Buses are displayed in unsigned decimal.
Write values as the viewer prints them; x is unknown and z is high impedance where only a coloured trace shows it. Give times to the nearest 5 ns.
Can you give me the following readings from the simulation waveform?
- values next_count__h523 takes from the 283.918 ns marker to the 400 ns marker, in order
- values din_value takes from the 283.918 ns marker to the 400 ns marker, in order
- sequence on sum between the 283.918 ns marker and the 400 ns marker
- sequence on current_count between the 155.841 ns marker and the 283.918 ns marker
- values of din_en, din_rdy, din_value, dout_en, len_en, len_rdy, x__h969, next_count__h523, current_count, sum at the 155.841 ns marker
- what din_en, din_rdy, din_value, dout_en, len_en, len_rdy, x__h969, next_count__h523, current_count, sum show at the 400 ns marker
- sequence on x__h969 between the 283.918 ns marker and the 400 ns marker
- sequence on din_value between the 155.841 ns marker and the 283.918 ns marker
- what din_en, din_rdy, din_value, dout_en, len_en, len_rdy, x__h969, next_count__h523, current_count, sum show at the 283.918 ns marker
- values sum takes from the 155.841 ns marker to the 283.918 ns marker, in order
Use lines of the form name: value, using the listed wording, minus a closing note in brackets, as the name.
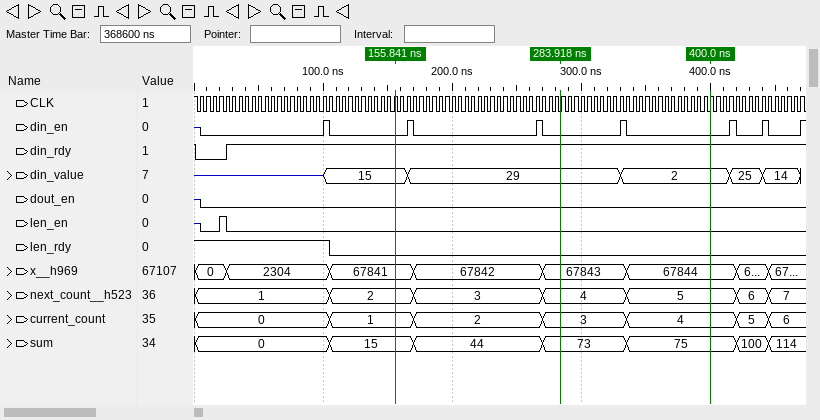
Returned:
values next_count__h523 takes from the 283.918 ns marker to the 400 ns marker, in order: 4, 5
values din_value takes from the 283.918 ns marker to the 400 ns marker, in order: 29, 2
sequence on sum between the 283.918 ns marker and the 400 ns marker: 73, 75
sequence on current_count between the 155.841 ns marker and the 283.918 ns marker: 1, 2, 3
values of din_en, din_rdy, din_value, dout_en, len_en, len_rdy, x__h969, next_count__h523, current_count, sum at the 155.841 ns marker: din_en=0, din_rdy=1, din_value=15, dout_en=0, len_en=0, len_rdy=0, x__h969=67841, next_count__h523=2, current_count=1, sum=15
what din_en, din_rdy, din_value, dout_en, len_en, len_rdy, x__h969, next_count__h523, current_count, sum show at the 400 ns marker: din_en=0, din_rdy=1, din_value=2, dout_en=0, len_en=0, len_rdy=0, x__h969=67844, next_count__h523=5, current_count=4, sum=75
sequence on x__h969 between the 283.918 ns marker and the 400 ns marker: 67843, 67844
sequence on din_value between the 155.841 ns marker and the 283.918 ns marker: 15, 29
what din_en, din_rdy, din_value, dout_en, len_en, len_rdy, x__h969, next_count__h523, current_count, sum show at the 283.918 ns marker: din_en=0, din_rdy=1, din_value=29, dout_en=0, len_en=0, len_rdy=0, x__h969=67843, next_count__h523=4, current_count=3, sum=73
values sum takes from the 155.841 ns marker to the 283.918 ns marker, in order: 15, 44, 73
